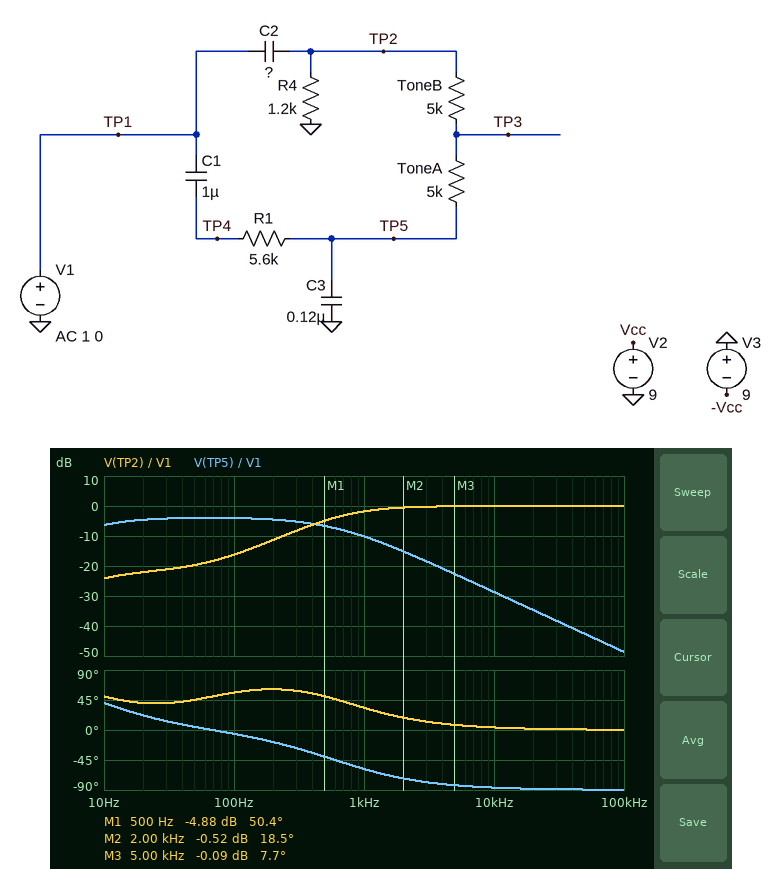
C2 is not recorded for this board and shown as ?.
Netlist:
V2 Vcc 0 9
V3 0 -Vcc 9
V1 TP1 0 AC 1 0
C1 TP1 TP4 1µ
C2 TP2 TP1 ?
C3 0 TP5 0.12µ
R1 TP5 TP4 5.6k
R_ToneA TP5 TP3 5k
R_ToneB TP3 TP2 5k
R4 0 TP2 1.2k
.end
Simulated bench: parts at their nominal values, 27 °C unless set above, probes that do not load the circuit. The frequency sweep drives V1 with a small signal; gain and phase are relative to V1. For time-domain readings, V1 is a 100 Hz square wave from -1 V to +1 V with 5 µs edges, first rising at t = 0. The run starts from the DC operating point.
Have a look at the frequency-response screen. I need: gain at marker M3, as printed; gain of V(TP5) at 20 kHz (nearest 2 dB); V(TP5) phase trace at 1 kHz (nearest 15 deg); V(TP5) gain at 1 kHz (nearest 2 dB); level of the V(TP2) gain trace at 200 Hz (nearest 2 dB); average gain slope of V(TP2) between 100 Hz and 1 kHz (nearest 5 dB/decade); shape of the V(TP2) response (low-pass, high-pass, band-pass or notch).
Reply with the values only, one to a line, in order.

-0.09 dB
-34 dB
-60 deg
-10 dB
-12 dB
15 dB/decade
high-pass
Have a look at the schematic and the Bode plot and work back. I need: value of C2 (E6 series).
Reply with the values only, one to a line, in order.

220 nF
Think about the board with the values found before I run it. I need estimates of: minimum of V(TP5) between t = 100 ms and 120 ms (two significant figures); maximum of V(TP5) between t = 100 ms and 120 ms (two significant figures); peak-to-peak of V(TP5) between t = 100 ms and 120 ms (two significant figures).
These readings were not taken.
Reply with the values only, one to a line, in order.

-670 mV
670 mV
1.3 V
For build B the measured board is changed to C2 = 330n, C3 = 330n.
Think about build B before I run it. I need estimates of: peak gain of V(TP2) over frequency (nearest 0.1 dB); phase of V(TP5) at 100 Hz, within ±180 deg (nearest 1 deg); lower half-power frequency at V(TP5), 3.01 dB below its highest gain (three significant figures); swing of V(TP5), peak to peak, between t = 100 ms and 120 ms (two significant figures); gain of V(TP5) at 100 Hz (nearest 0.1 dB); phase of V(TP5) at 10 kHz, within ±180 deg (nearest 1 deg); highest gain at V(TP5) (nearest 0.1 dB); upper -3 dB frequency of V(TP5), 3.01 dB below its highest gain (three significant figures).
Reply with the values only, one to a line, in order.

0 dB
-23 deg
7.45 Hz
1.1 V
-5.9 dB
-88 deg
-4.9 dB
188 Hz
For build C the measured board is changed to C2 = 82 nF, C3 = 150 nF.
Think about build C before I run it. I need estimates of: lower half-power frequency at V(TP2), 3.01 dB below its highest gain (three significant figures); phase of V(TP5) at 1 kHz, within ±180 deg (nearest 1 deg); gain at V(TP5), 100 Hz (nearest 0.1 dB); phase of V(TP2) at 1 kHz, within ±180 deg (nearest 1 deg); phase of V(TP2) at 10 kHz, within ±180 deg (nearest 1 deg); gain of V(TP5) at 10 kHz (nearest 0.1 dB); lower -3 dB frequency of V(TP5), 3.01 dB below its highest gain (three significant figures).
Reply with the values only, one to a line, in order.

1.86 kHz
-61 deg
-4.5 dB
60 deg
10 deg
-30.7 dB
8.39 Hz
